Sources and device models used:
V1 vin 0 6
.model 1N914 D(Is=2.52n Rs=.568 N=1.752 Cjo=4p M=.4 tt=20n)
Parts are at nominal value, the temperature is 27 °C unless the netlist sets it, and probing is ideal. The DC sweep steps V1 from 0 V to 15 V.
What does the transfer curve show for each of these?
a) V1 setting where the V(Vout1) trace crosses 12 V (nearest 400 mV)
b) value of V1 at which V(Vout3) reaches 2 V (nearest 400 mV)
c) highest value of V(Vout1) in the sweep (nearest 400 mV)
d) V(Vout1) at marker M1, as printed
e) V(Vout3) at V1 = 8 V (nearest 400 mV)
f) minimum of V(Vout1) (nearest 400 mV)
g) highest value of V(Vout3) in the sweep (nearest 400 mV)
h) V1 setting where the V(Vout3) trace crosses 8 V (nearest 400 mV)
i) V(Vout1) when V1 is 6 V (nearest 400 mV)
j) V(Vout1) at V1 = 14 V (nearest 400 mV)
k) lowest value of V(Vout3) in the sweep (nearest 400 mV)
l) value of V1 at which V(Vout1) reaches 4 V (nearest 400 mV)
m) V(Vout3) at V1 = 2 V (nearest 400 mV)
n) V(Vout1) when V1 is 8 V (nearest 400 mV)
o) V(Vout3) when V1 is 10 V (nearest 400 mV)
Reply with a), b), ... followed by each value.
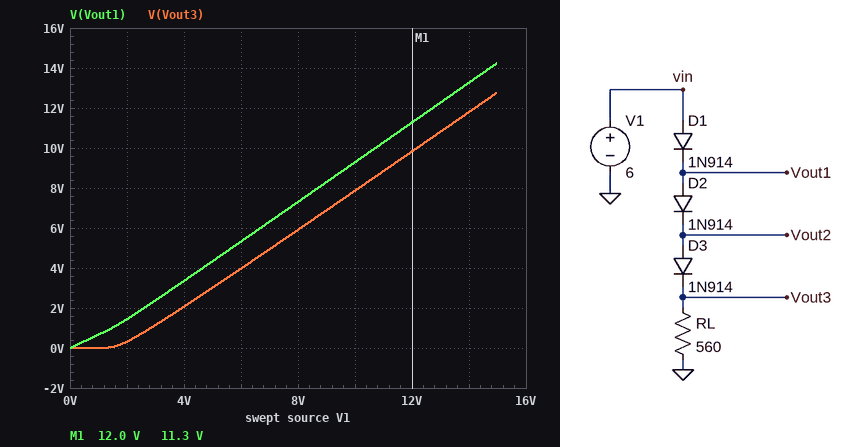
a) 12.8 V
b) 4.0 V
c) 14.4 V
d) 11.3 V
e) 6.0 V
f) 0 V
g) 12.8 V
h) 10.0 V
i) 5.2 V
j) 13.2 V
k) 0 V
l) 4.8 V
m) 400 mV
n) 7.2 V
o) 8.0 V
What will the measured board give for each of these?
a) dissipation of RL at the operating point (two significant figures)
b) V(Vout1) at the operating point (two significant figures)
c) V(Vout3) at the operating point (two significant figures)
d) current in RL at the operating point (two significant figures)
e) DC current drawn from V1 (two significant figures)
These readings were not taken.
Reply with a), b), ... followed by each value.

a) 28 mW
b) 5.3 V
c) 4.0 V
d) 7.1 mA
e) 7.1 mA
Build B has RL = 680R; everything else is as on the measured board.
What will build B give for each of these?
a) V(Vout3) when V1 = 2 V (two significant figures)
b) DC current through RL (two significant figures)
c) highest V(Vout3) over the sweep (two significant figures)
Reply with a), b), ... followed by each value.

a) 340 mV
b) 5.9 mA
c) 13 V
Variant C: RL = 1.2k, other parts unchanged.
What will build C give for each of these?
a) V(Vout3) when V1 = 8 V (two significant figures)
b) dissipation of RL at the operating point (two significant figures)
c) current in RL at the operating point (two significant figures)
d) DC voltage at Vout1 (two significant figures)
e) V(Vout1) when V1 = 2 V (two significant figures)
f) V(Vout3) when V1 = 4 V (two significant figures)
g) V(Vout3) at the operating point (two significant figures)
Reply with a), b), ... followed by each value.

a) 6.0 V
b) 14 mW
c) 3.4 mA
d) 5.4 V
e) 1.5 V
f) 2.2 V
g) 4.1 V
